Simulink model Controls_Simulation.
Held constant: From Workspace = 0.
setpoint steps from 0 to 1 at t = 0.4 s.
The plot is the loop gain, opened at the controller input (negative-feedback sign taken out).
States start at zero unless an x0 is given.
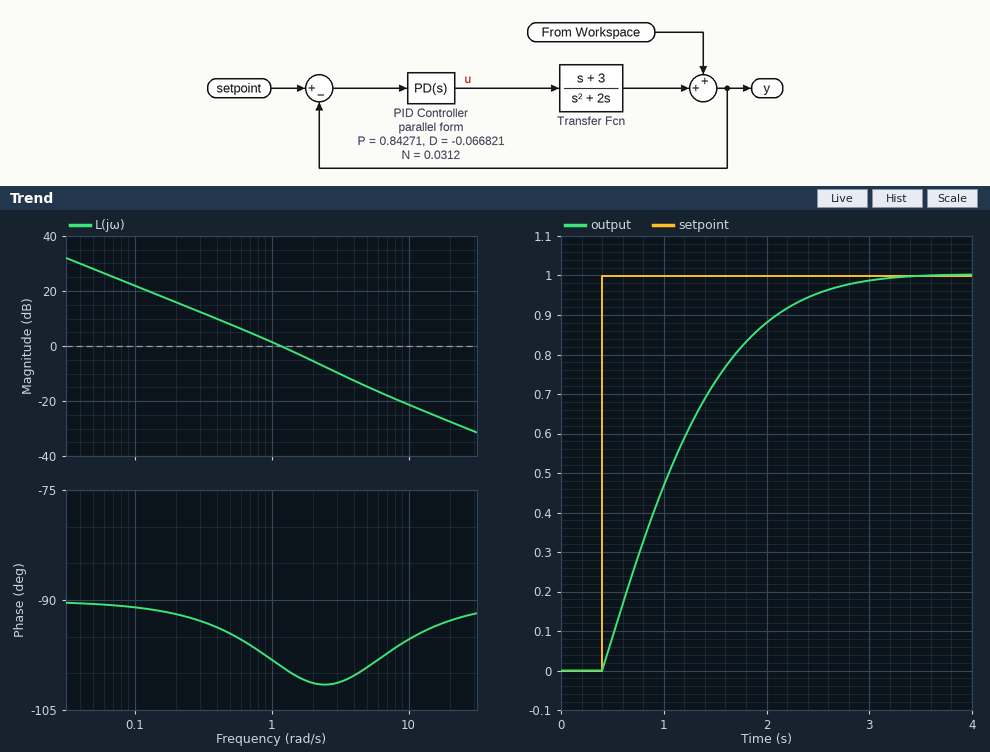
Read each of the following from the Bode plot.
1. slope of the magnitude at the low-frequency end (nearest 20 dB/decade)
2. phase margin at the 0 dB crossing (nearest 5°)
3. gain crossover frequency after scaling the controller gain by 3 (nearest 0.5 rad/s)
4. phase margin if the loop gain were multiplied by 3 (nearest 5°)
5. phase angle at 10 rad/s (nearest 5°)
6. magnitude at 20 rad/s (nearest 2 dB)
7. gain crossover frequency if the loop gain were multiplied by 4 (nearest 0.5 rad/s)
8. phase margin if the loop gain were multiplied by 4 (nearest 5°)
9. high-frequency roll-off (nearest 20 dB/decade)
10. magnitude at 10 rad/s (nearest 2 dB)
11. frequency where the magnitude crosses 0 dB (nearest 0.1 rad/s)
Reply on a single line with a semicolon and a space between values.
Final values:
-20 dB/decade; 80°; 3.0 rad/s; 80°; -95°; -28 dB; 4.0 rad/s; 80°; -20 dB/decade; -22 dB; 1.2 rad/s
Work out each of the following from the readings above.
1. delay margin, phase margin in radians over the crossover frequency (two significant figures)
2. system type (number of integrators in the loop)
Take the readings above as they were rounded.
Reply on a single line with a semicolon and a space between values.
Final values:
1.2 s; 1
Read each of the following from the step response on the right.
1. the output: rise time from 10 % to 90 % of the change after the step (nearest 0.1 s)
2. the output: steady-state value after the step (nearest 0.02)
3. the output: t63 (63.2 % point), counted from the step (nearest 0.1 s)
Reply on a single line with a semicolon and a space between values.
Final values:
1.6 s; 1.00; 0.9 s
